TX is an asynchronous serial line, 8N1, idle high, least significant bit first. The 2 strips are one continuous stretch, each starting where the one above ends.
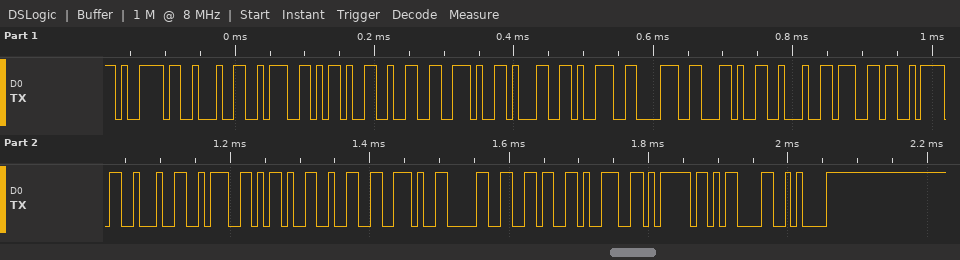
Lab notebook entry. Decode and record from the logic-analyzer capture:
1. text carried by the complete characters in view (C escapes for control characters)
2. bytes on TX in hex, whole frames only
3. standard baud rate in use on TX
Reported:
"y\":-2.198,\"gz\":-2.069}\r\n"
0x79 0x22 0x3A 0x2D 0x32 0x2E 0x31 0x39 0x38 0x2C 0x22 0x67 0x7A 0x22 0x3A 0x2D 0x32 0x2E 0x30 0x36 0x39 0x7D 0x0D 0x0A
115200 baud
